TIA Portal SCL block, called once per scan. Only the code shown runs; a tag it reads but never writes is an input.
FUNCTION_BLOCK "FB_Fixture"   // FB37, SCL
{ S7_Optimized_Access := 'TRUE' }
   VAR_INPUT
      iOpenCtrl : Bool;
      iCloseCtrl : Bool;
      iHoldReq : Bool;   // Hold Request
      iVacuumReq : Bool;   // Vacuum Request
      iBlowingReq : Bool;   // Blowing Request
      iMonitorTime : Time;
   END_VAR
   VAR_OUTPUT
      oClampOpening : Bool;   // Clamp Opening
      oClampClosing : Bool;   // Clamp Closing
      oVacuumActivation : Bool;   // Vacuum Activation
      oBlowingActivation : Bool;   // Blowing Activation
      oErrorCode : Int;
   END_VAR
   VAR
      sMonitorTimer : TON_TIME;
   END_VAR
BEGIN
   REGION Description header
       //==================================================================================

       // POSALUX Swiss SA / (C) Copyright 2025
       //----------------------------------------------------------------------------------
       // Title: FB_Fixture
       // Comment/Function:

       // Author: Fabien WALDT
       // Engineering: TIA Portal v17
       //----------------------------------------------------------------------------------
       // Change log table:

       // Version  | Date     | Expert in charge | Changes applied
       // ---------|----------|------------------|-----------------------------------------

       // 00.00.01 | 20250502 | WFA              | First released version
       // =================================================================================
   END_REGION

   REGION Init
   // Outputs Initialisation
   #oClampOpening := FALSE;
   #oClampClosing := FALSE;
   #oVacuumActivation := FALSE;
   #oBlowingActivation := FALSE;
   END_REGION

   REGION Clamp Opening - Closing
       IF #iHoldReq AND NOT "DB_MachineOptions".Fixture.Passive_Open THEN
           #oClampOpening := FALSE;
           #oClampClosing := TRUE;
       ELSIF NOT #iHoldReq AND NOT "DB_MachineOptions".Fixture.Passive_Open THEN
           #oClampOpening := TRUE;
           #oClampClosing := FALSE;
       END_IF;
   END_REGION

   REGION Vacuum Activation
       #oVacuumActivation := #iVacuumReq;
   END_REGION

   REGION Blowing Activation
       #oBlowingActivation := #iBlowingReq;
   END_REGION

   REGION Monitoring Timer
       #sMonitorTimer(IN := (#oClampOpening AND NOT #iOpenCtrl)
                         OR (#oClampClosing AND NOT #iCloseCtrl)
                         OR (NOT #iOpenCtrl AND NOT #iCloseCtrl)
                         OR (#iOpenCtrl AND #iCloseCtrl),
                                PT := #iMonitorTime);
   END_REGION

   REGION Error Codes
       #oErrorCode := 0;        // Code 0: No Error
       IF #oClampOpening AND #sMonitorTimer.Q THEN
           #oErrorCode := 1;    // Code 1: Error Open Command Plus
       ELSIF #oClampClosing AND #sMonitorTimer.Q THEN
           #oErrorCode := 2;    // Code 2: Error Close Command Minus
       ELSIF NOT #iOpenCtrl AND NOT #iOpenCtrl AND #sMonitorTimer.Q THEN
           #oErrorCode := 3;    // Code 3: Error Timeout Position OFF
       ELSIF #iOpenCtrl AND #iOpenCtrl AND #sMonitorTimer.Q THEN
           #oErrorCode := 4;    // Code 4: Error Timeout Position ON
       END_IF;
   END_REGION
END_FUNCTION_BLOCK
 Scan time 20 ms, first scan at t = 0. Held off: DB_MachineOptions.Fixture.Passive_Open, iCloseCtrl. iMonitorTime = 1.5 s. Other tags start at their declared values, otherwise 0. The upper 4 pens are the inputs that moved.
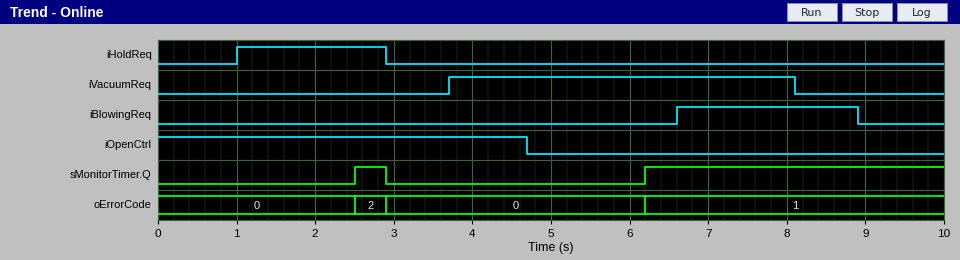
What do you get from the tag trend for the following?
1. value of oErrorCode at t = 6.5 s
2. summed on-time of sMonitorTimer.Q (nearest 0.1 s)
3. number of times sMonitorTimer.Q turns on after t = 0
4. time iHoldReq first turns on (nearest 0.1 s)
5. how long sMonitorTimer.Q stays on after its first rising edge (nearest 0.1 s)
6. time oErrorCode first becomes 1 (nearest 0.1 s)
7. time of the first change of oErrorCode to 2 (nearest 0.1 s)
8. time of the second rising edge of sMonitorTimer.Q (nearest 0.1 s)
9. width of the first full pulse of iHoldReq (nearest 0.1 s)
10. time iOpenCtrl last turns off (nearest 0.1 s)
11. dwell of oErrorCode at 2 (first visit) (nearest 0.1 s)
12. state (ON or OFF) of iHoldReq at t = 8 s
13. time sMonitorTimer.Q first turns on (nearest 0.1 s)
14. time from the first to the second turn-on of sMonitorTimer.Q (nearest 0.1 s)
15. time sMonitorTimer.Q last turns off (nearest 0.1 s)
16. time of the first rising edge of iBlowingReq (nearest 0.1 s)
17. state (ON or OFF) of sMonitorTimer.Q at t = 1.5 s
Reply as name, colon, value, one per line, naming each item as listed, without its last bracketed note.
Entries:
value of oErrorCode at t = 6.5 s: 1
summed on-time of sMonitorTimer.Q: 4.2 s
number of times sMonitorTimer.Q turns on after t = 0: 2
time iHoldReq first turns on: 1.0 s
how long sMonitorTimer.Q stays on after its first rising edge: 0.4 s
time oErrorCode first becomes 1: 6.2 s
time of the first change of oErrorCode to 2: 2.5 s
time of the second rising edge of sMonitorTimer.Q: 6.2 s
width of the first full pulse of iHoldReq: 1.9 s
time iOpenCtrl last turns off: 4.7 s
dwell of oErrorCode at 2 (first visit): 0.4 s
state (ON or OFF) of iHoldReq at t = 8 s: OFF
time sMonitorTimer.Q first turns on: 2.5 s
time from the first to the second turn-on of sMonitorTimer.Q: 3.7 s
time sMonitorTimer.Q last turns off: 2.9 s
time of the first rising edge of iBlowingReq: 6.6 s
state (ON or OFF) of sMonitorTimer.Q at t = 1.5 s: OFF
